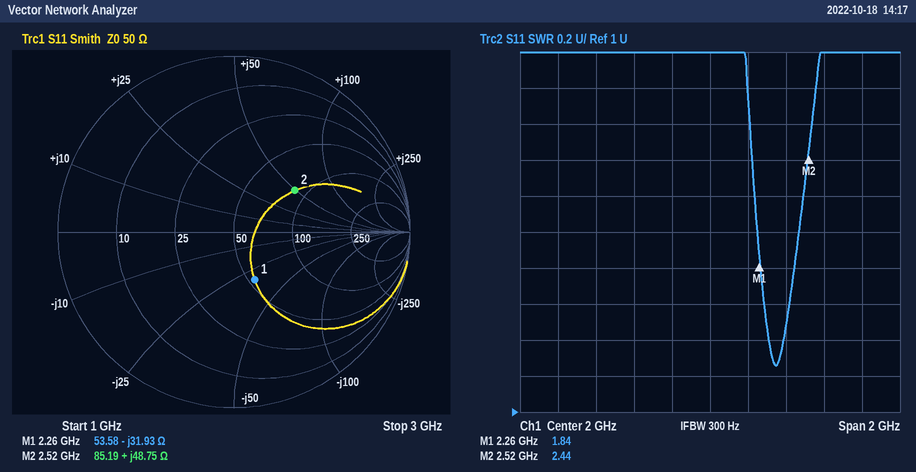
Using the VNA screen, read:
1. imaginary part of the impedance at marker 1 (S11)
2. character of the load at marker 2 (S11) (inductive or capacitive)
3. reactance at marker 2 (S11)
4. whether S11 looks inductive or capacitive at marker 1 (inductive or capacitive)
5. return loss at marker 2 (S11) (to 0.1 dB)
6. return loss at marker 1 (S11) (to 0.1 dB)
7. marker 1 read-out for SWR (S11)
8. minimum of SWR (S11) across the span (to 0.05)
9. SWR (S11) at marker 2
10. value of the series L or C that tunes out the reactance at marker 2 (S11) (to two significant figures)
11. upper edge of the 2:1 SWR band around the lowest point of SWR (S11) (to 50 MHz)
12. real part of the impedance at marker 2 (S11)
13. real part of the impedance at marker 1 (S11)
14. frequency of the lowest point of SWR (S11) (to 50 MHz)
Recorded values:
-31.93 Ω
inductive
+48.75 Ω
capacitive
7.6 dB
10.6 dB
1.84
1.25
2.44
1.3 pF
2.45 GHz
85.19 Ω
53.58 Ω
2.35 GHz
